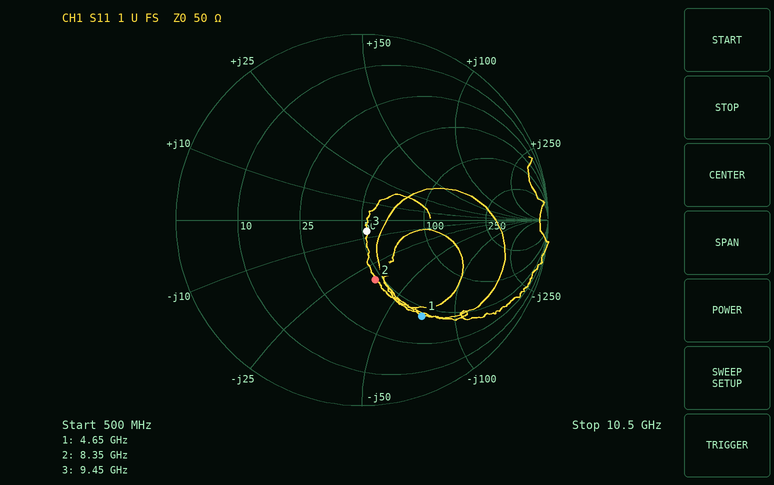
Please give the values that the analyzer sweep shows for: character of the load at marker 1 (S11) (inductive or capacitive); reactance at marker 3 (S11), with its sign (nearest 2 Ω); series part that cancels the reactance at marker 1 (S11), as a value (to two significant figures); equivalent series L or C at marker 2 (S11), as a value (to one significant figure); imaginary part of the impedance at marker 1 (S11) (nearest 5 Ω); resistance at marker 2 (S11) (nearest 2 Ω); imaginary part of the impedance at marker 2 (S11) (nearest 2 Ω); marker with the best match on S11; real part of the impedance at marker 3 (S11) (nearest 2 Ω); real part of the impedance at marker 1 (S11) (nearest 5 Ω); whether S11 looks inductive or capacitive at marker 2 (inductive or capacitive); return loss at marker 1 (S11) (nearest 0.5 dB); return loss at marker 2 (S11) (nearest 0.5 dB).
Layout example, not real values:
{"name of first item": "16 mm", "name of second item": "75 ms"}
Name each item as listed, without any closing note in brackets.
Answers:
{"character of the load at marker 1 (S11)": "capacitive", "reactance at marker 3 (S11), with its sign": "-6 Ω", "series part that cancels the reactance at marker 1 (S11), as a value": "2.4 nH", "equivalent series L or C at marker 2 (S11), as a value": "600 fF", "imaginary part of the impedance at marker 1 (S11)": "-70 Ω", "resistance at marker 2 (S11)": "46 Ω", "imaginary part of the impedance at marker 2 (S11)": "-34 Ω", "marker with the best match on S11": "marker 3", "real part of the impedance at marker 3 (S11)": "52 Ω", "real part of the impedance at marker 1 (S11)": "45 Ω", "whether S11 looks inductive or capacitive at marker 2": "capacitive", "return loss at marker 1 (S11)": "4.5 dB", "return loss at marker 2 (S11)": "9.5 dB"}
